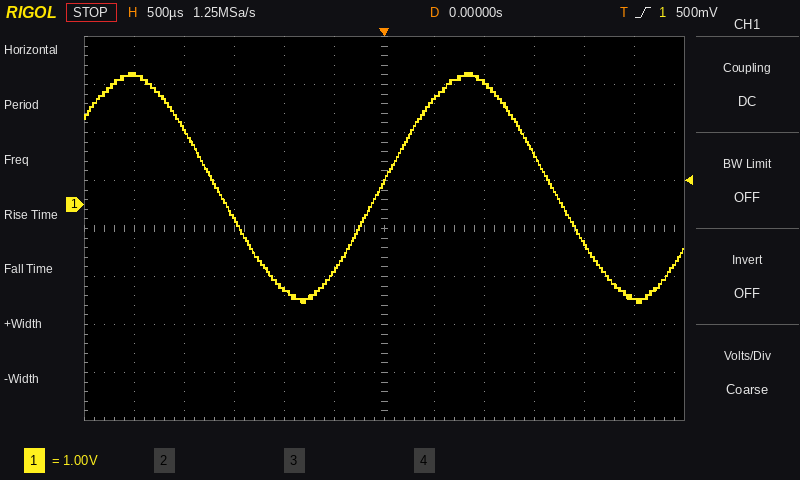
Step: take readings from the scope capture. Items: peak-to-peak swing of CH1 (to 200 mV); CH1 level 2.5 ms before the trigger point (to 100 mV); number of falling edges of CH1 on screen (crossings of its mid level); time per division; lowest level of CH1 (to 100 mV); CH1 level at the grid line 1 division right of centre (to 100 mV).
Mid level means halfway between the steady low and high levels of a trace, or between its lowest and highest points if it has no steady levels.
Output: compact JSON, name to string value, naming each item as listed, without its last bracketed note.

{"peak-to-peak swing of CH1": "4.8 V", "CH1 level 2.5 ms before the trigger point": "2.7 V", "number of falling edges of CH1 on screen": "2", "time per division": "500 µs", "lowest level of CH1": "-2.0 V", "CH1 level at the grid line 1 division right of centre": "2.2 V"}
